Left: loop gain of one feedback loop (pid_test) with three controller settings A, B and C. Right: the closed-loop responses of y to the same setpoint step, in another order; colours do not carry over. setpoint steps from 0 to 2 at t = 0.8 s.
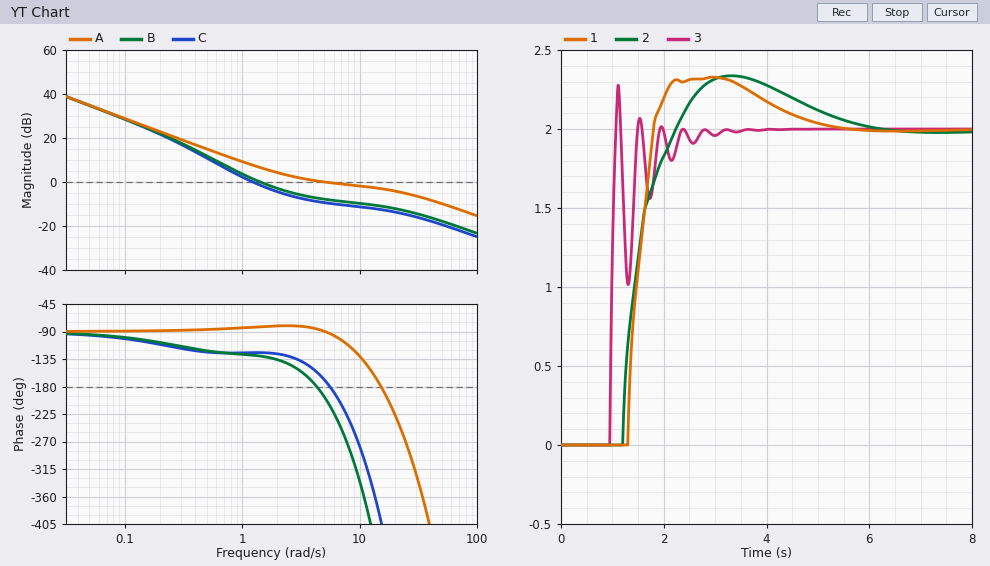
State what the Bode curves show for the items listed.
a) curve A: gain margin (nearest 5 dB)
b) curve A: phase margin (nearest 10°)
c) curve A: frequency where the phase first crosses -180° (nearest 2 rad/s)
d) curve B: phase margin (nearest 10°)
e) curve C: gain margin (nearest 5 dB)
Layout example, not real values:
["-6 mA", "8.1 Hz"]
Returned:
["5 dB", "90°", "16 rad/s", "50°", "10 dB"]
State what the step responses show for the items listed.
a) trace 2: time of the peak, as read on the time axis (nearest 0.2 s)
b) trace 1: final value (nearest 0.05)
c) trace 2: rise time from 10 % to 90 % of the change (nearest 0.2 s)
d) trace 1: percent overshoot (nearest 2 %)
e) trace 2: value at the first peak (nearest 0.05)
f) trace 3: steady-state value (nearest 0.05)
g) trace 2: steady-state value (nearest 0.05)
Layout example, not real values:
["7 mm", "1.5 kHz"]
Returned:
["3.4 s", "2.00", "0.8 s", "16 %", "2.35", "2.00", "2.00"]
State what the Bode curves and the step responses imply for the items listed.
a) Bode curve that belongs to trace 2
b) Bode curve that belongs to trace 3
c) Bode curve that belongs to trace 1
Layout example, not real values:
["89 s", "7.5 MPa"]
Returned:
["C", "A", "B"]
